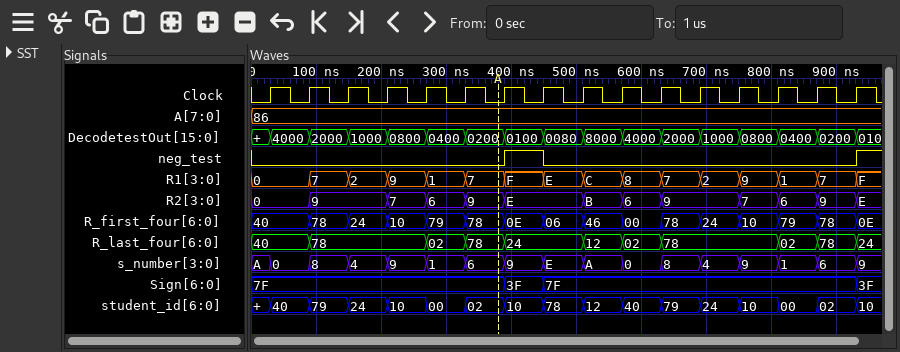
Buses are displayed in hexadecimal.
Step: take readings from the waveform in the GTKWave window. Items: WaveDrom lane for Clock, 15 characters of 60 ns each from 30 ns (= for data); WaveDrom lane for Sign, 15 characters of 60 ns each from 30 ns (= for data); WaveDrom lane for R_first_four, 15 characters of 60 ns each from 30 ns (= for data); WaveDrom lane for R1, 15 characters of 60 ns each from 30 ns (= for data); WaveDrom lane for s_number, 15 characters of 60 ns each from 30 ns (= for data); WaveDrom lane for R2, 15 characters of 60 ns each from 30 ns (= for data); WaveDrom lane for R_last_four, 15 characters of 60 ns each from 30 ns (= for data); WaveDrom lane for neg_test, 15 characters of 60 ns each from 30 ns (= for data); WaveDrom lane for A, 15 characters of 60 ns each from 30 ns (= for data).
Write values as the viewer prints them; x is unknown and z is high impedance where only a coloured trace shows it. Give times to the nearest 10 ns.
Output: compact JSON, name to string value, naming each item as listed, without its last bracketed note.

{"WaveDrom lane for Clock, 15 characters of 60 ns each from 30 ns": "{name: 'Clock', wave: 'p..............'}", "WaveDrom lane for Sign, 15 characters of 60 ns each from 30 ns": "{name: 'Sign', wave: '=.....==.......', data: '7F 3F 7F'}", "WaveDrom lane for R_first_four, 15 characters of 60 ns each from 30 ns": "{name: 'R_first_four', wave: '===============', data: '40 78 24 10 79 78 0E 06 46 00 78 24 10 79 78'}", "WaveDrom lane for R1, 15 characters of 60 ns each from 30 ns": "{name: 'R1', wave: '===============', data: '0 7 2 9 1 7 F E C 8 7 2 9 1 7'}", "WaveDrom lane for s_number, 15 characters of 60 ns each from 30 ns": "{name: 's_number', wave: '===============', data: '0 8 4 9 1 6 9 E A 0 8 4 9 1 6'}", "WaveDrom lane for R2, 15 characters of 60 ns each from 30 ns": "{name: 'R2', wave: '==.====.===.===', data: '0 9 7 6 9 E B 6 9 7 6 9'}", "WaveDrom lane for R_last_four, 15 characters of 60 ns each from 30 ns": "{name: 'R_last_four', wave: '==..===.===..==', data: '40 78 02 78 24 12 02 78 02 78'}", "WaveDrom lane for neg_test, 15 characters of 60 ns each from 30 ns": "{name: 'neg_test', wave: '0.....10.......'}", "WaveDrom lane for A, 15 characters of 60 ns each from 30 ns": "{name: 'A', wave: '=..............', data: '86'}"}
